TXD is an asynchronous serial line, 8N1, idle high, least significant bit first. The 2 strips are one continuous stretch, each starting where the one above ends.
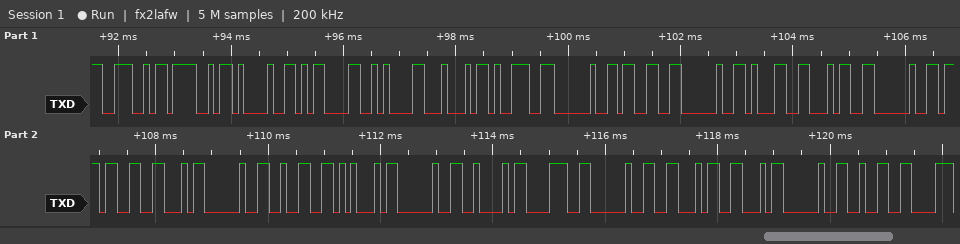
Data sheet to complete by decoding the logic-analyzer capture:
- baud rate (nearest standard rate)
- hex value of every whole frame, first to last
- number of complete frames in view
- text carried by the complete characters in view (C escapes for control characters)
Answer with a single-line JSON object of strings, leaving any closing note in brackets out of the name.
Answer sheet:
{"baud rate": "9600 baud", "hex value of every whole frame, first to last": "4E 4F 21 0D 0A 44 39 20 33 20 31 34 20 37 46 20 32 45 20 42 38 20 46 46 20 32", "number of complete frames in view": "26", "text carried by the complete characters in view": "\"NO!\\r\\nD9 3 14 7F 2E B8 FF 2\""}
